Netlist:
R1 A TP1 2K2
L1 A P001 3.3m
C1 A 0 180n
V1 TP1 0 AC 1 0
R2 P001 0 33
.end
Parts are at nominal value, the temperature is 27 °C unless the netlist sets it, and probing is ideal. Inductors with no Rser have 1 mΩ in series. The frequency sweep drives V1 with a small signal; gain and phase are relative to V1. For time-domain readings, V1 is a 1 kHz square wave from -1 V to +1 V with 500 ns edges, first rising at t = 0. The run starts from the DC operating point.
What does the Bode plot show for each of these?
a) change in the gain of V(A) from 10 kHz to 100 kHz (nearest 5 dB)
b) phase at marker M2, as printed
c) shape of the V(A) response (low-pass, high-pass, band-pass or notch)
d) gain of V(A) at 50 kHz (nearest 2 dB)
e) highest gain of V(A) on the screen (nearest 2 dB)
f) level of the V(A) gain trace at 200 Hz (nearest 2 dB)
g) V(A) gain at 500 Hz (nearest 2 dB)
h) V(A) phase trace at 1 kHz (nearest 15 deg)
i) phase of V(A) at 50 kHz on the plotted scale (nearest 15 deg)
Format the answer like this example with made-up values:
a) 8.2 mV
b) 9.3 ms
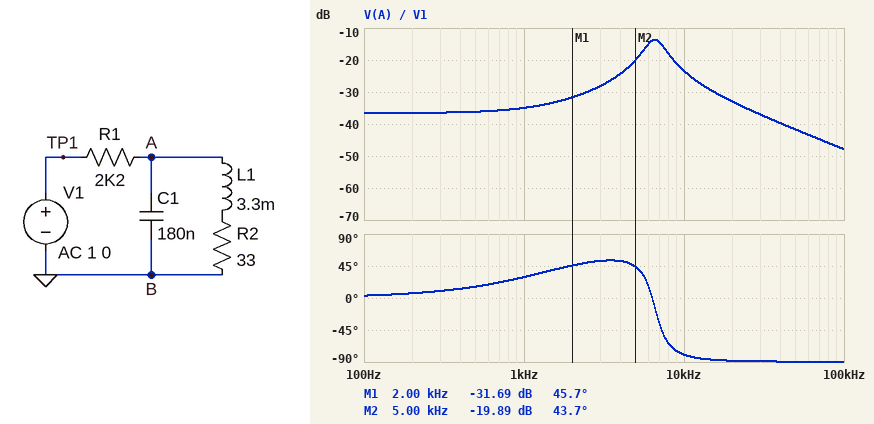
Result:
a) -25 dB
b) 43.7 deg
c) band-pass
d) -42 dB
e) -14 dB
f) -36 dB
g) -36 dB
h) 30 deg
i) -90 deg
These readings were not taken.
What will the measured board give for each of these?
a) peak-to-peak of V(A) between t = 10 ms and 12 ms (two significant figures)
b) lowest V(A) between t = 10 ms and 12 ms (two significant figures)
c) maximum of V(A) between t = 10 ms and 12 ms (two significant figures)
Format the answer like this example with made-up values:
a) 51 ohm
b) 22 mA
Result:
a) 220 mV
b) -110 mV
c) 110 mV
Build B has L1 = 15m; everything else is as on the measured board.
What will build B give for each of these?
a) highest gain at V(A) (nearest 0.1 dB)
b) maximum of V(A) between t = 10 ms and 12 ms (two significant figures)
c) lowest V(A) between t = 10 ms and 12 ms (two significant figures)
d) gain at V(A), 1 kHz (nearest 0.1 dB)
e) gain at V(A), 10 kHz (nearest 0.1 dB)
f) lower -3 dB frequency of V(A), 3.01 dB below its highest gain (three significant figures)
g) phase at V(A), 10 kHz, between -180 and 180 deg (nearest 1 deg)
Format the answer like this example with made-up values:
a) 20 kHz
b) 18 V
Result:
a) -5.4 dB
b) 320 mV
c) -320 mV
d) -26.1 dB
e) -27.1 dB
f) 2.73 kHz
g) -87 deg
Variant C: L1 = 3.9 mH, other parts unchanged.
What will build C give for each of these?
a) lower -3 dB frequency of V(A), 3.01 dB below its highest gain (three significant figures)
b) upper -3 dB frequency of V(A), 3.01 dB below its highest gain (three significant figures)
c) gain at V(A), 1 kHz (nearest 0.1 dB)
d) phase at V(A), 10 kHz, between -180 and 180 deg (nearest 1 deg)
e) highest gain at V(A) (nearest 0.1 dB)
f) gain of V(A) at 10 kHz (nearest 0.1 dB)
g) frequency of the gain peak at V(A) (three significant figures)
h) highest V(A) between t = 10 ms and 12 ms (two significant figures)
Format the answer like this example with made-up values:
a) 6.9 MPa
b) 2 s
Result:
a) 5.23 kHz
b) 6.98 kHz
c) -34.5 dB
d) -82 deg
e) -12.6 dB
f) -24.2 dB
g) 6.05 kHz
h) 110 mV
